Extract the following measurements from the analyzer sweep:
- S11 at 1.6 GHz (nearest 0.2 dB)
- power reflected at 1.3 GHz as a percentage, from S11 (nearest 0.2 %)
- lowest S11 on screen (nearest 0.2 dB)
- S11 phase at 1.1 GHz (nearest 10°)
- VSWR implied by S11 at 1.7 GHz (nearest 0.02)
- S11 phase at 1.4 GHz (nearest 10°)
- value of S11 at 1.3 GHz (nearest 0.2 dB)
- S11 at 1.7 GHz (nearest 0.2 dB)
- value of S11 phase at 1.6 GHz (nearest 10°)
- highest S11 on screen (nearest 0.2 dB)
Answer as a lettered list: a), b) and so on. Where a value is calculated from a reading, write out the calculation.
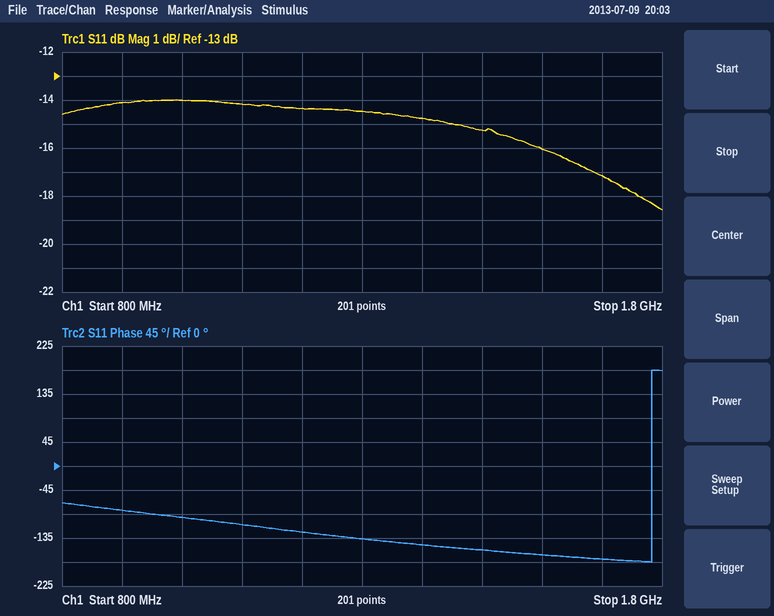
a) -16.0 dB
b) 10^(-14.4/10) ≈ 3.6 %
c) -18.6 dB
d) -110°
e) |Γ| = 10^(-17.2/20) = 0.1380; VSWR = (1 + 0.1380)/(1 − 0.1380) ≈ 1.32
f) -150°
g) -14.4 dB
h) -17.2 dB
i) -170°
j) -14.0 dB
